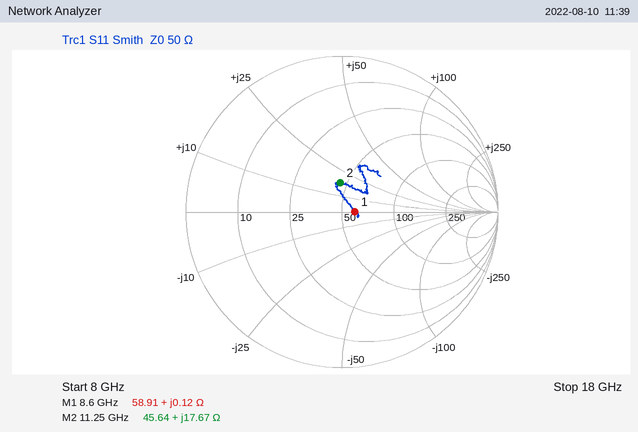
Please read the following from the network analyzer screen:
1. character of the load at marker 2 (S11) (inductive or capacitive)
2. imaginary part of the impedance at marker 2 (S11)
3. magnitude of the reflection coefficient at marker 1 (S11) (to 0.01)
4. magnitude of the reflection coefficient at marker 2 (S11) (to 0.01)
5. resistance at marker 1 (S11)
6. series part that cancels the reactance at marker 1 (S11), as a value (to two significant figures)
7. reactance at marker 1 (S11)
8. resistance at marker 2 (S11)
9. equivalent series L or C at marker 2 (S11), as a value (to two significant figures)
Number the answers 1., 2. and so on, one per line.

1. inductive
2. +17.67 Ω
3. 0.08
4. 0.19
5. 58.91 Ω
6. 150 pF
7. +0.12 Ω
8. 45.64 Ω
9. 250 pH
